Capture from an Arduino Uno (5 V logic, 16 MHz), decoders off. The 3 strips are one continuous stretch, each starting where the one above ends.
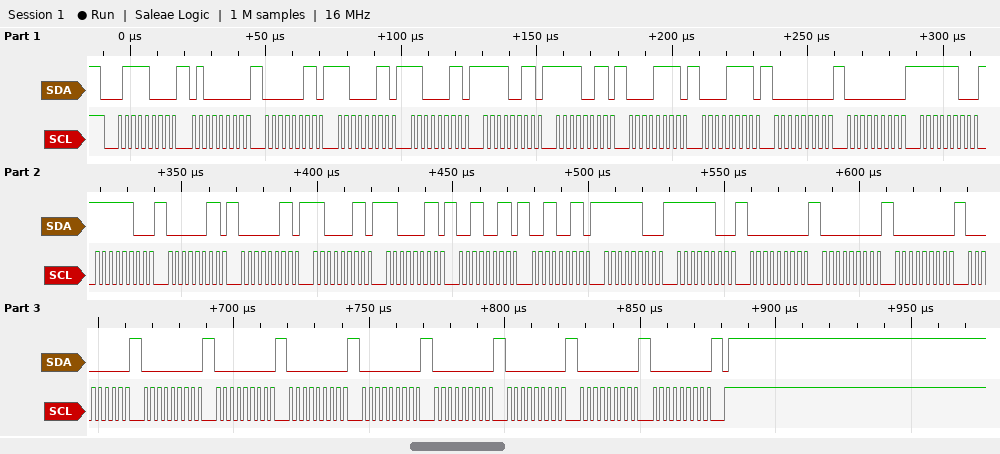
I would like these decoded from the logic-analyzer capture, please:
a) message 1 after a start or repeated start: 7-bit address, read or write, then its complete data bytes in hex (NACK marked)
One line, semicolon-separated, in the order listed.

0x3C write: 40 03 C3 C3 F3 F3 0F 0F 00 00 FC FC 03 03 C3 C3 33 33 FC FC 00 00 00 00 00 00 00 00 00 00 00 00
